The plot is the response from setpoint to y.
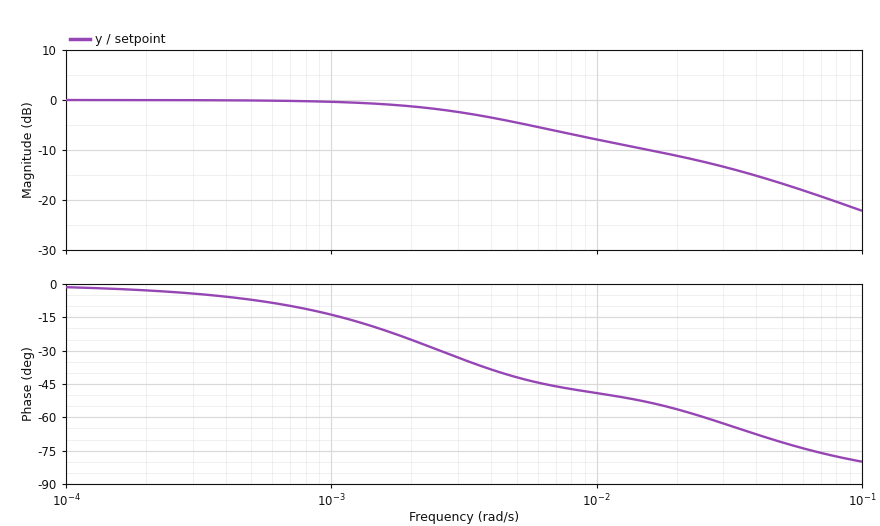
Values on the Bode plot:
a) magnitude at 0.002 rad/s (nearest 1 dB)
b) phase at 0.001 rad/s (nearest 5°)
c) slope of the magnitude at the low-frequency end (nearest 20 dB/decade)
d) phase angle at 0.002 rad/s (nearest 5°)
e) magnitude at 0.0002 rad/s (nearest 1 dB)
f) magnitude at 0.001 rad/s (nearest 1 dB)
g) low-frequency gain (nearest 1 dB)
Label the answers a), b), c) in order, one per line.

a) -1 dB
b) -15°
c) 0 dB/decade
d) -25°
e) 0 dB
f) 0 dB
g) 0 dB
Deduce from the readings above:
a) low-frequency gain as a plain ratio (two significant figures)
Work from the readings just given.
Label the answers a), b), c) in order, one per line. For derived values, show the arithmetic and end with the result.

a) 10^(0 / 20) = 1.0
